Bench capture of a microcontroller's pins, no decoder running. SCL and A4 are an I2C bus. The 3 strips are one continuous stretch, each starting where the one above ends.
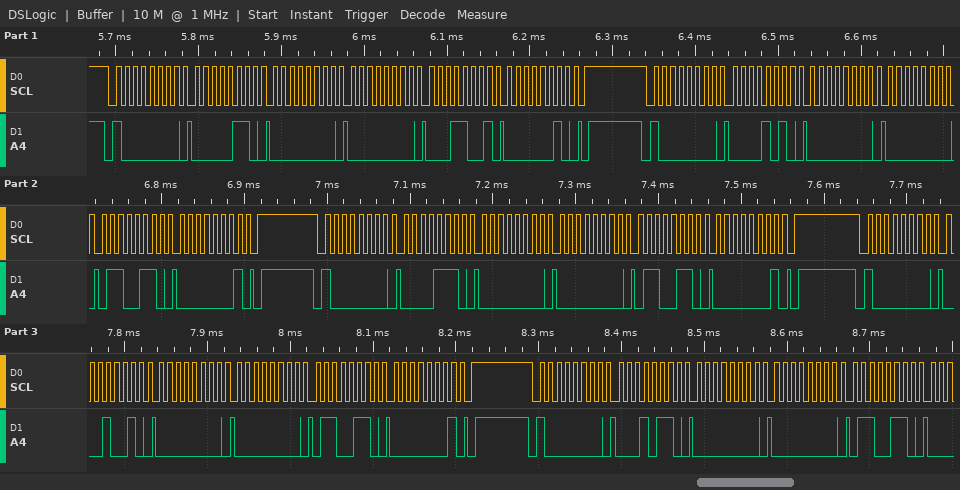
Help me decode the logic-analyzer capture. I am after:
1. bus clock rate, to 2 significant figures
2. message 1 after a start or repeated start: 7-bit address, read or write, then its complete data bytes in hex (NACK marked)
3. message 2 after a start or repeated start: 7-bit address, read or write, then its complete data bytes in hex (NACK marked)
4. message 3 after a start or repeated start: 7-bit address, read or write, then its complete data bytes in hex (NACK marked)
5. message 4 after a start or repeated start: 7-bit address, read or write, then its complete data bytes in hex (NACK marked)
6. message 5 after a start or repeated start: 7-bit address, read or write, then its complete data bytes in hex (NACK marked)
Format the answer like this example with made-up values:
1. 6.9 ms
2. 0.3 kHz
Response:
1. 100 kHz
2. 0x40 write: 06 00 00 19 02
3. 0x40 write: 0A 00 00 66 01
4. 0x40 write: 0E 00 00 66 01
5. 0x40 write: 12 00 00 66 01
6. 0x40 write: 16 00 00 66
